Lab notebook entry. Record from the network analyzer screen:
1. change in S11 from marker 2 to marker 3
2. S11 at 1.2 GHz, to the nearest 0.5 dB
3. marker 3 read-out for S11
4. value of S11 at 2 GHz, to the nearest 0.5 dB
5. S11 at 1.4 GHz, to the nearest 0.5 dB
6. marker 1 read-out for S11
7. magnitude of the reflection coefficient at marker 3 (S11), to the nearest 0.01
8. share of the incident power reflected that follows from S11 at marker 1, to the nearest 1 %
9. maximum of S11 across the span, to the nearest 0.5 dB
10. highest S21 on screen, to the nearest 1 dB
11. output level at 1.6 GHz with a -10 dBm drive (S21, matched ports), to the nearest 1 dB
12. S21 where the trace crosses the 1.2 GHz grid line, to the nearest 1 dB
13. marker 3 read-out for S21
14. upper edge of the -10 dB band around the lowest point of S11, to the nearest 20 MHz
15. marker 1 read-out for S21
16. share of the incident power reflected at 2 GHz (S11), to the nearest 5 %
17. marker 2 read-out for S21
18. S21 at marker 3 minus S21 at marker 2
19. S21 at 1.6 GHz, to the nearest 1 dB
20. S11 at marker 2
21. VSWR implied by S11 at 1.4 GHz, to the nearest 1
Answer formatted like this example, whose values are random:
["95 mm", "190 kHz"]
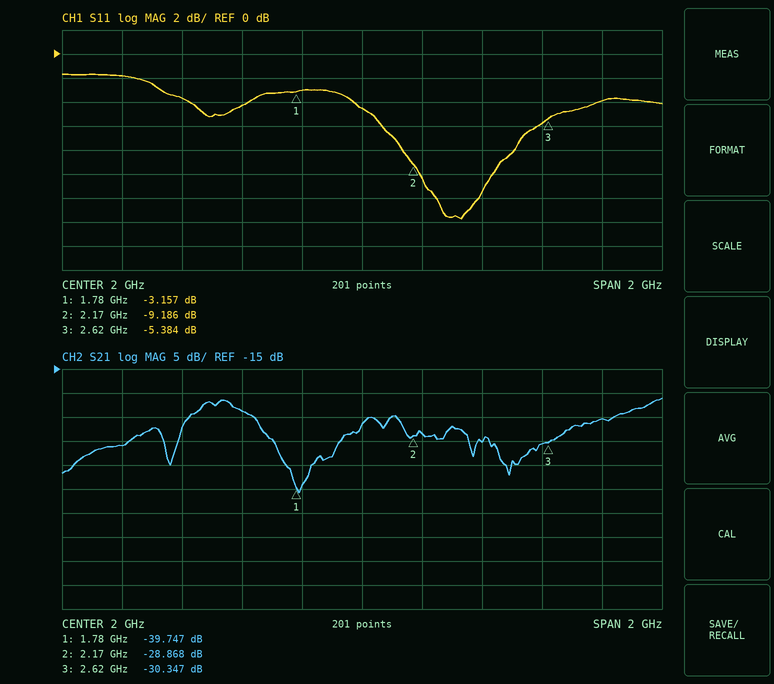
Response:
["3.802 dB", "-2.0 dB", "-5.384 dB", "-4.5 dB", "-3.5 dB", "-3.157 dB", "0.54", "48 %", "-1.5 dB", "-21 dB", "-34 dBm", "-31 dB", "-30.347 dB", "2.44 GHz", "-39.747 dB", "35 %", "-28.868 dB", "-1.479 dB", "-24 dB", "-9.186 dB", "5"]
